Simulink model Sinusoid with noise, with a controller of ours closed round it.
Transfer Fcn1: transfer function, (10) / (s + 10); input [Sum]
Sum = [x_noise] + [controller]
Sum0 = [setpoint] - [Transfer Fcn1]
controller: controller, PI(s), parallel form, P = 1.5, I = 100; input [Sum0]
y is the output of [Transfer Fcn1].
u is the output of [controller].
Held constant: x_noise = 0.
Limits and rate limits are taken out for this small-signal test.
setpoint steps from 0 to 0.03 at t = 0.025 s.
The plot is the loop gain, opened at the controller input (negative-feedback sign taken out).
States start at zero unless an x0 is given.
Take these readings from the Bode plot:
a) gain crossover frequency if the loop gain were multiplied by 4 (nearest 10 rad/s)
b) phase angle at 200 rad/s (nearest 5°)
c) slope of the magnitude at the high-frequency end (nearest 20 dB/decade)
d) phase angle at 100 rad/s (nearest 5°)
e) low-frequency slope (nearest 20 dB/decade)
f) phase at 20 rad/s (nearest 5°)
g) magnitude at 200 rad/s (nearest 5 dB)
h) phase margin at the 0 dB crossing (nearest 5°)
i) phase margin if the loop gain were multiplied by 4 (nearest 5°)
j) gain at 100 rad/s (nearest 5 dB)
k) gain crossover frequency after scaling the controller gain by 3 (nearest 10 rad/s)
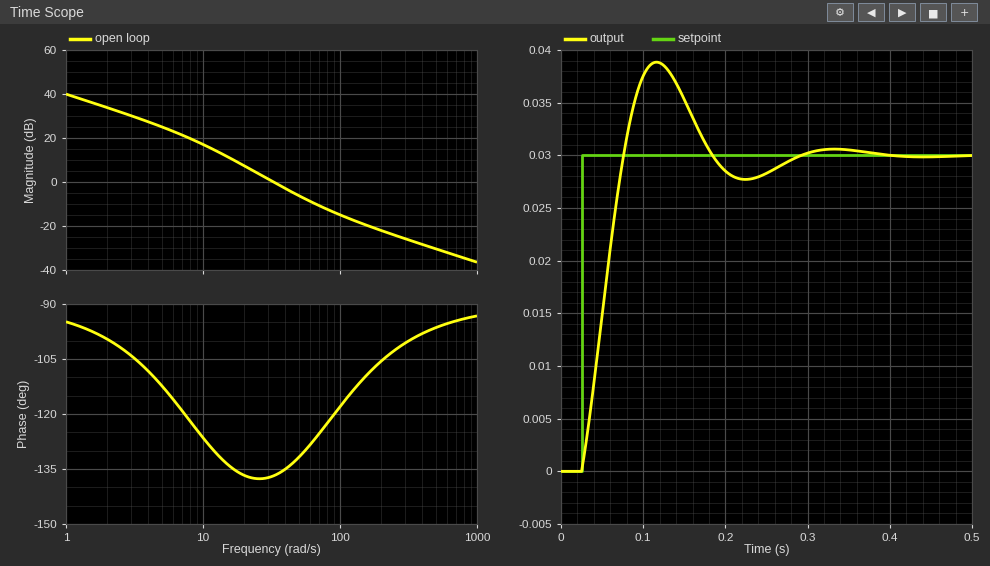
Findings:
80 rad/s
-105°
-20 dB/decade
-120°
-20 dB/decade
-135°
-20 dB
45°
55°
-15 dB
60 rad/s
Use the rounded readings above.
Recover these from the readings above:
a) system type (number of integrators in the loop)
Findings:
1
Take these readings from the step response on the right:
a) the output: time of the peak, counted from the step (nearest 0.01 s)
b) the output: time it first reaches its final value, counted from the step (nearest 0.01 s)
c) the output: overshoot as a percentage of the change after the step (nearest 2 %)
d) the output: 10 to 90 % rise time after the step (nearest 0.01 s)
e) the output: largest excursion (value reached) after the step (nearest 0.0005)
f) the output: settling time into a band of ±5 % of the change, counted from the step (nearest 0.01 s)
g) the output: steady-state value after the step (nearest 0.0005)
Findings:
0.09 s
0.05 s
30 %
0.04 s
0.0390
0.23 s
0.0300
